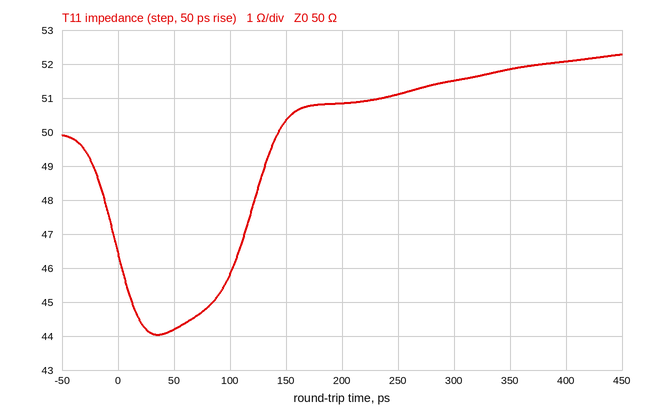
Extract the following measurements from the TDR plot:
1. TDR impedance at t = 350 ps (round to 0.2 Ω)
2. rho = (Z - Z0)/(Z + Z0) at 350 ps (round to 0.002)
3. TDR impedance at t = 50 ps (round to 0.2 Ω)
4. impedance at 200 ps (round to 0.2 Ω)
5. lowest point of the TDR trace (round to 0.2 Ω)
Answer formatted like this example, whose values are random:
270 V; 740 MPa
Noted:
51.8 Ω; +0.018; 44.2 Ω; 50.8 Ω; 44.0 Ω
